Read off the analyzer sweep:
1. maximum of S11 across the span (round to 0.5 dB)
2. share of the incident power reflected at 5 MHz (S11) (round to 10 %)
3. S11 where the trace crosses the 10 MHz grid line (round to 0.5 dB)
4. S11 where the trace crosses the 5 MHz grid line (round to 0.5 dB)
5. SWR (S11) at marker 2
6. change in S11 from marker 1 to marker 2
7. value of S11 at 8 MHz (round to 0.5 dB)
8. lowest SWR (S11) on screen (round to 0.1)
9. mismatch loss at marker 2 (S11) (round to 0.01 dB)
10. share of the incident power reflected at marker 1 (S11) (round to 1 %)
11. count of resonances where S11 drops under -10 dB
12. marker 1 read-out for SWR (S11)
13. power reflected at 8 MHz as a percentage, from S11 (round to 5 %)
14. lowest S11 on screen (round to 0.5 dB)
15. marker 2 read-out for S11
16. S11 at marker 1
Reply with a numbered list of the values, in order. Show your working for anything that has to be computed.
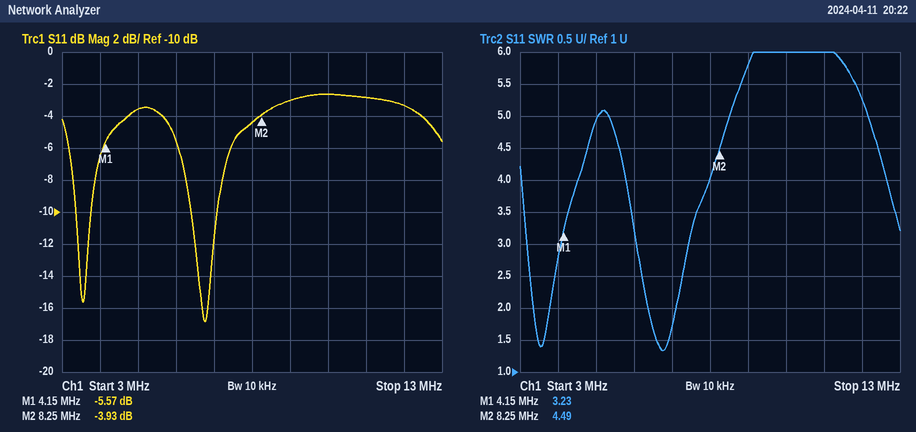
1. -2.5 dB
2. 10^(-3.5/10) ≈ 44.7 %, so 40 % to the nearest 10 %
3. -2.5 dB
4. -3.5 dB
5. 4.49
6. -3.93 − (-5.57) = 1.64 dB
7. -4.5 dB
8. 1.3
9. −10 log10(1 − 10^(-3.93/10)) ≈ 2.25 dB
10. 10^(-5.57/10) ≈ 28 %
11. 2
12. 3.23
13. 10^(-4.5/10) ≈ 35 %
14. -17.0 dB
15. -3.93 dB
16. -5.57 dB
